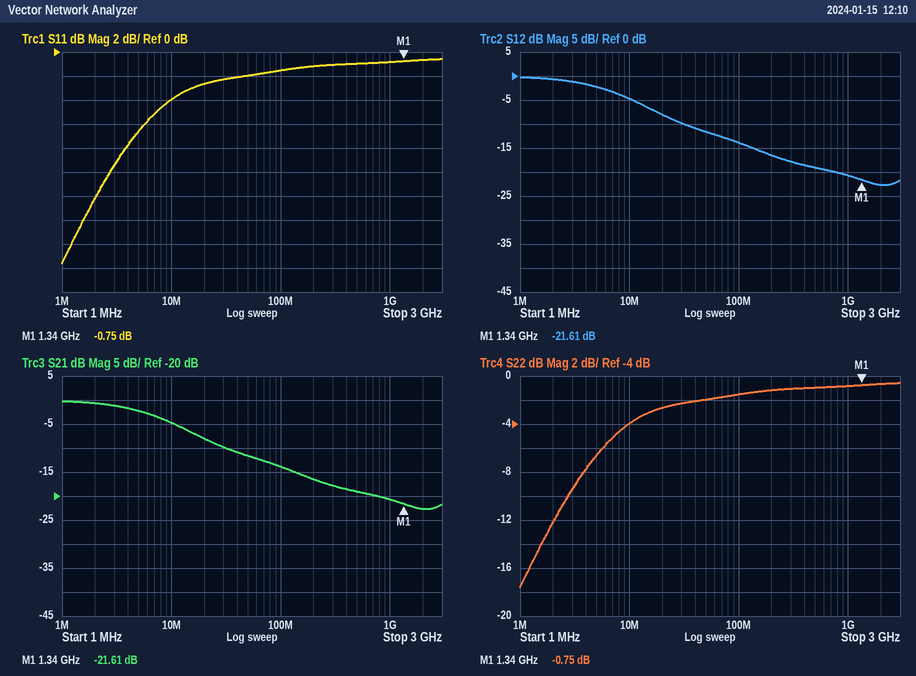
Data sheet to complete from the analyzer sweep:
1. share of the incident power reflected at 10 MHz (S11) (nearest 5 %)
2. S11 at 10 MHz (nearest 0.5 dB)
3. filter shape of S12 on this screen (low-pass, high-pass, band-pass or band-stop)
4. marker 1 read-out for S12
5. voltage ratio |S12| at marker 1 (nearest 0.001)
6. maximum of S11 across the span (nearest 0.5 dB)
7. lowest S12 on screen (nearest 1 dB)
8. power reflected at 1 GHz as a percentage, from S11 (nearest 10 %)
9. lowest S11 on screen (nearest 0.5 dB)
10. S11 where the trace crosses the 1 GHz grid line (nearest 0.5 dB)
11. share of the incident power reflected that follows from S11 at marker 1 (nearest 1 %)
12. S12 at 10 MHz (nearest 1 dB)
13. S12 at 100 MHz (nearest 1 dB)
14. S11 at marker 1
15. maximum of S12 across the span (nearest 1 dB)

40 %
-4.0 dB
low-pass
-21.61 dB
0.083
-0.5 dB
-23 dB
80 %
-17.5 dB
-1.0 dB
84 %
-5 dB
-14 dB
-0.75 dB
0 dB
